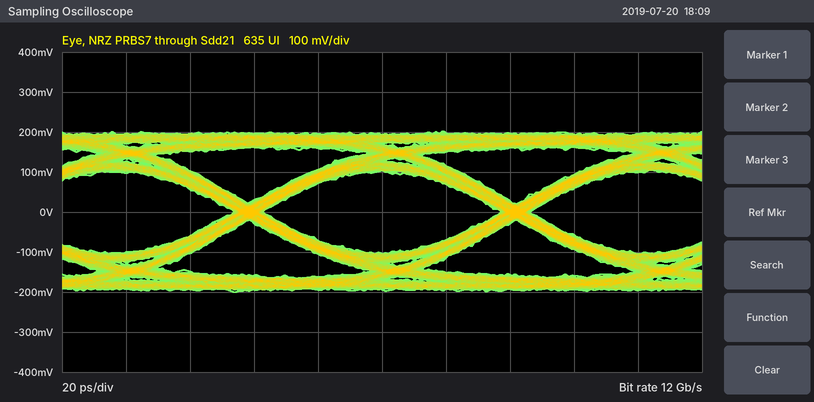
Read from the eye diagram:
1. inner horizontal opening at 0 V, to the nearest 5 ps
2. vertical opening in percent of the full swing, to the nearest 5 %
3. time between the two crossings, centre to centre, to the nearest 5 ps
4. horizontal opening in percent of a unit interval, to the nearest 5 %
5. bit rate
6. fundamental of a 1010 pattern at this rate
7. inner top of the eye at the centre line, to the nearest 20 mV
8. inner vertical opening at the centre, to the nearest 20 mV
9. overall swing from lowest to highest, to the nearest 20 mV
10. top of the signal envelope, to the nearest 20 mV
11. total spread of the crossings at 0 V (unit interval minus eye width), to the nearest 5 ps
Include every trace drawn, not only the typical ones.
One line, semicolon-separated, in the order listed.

75 ps; 50 %; 85 ps; 90 %; 12 Gb/s; 6 GHz; 100 mV; 200 mV; 400 mV; 200 mV; 10 ps
